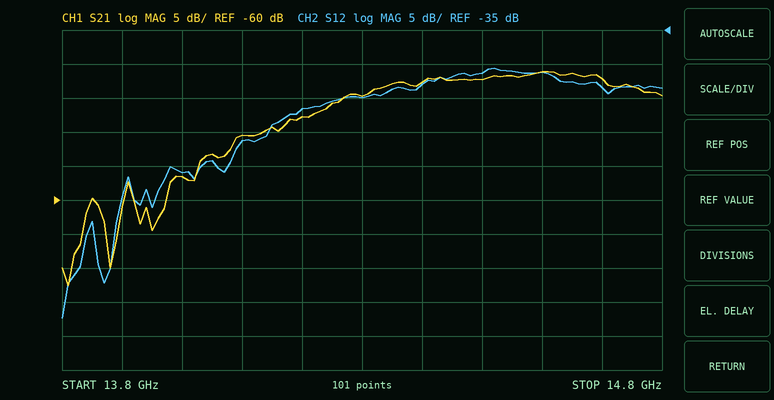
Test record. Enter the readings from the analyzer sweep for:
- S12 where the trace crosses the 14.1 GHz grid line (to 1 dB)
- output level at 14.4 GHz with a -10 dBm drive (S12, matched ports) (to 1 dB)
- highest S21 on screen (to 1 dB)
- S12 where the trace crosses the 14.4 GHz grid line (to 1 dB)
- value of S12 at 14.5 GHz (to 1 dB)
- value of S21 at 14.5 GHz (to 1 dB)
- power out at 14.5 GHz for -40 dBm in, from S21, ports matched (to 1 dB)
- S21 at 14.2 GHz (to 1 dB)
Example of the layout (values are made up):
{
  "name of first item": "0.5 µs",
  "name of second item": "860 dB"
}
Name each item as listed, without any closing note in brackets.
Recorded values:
{
  "S12 where the trace crosses the 14.1 GHz grid line": "-51 dB",
  "output level at 14.4 GHz with a -10 dBm drive (S12, matched ports)": "-53 dBm",
  "highest S21 on screen": "-41 dB",
  "S12 where the trace crosses the 14.4 GHz grid line": "-43 dB",
  "value of S12 at 14.5 GHz": "-41 dB",
  "value of S21 at 14.5 GHz": "-42 dB",
  "power out at 14.5 GHz for -40 dBm in, from S21, ports matched": "-82 dBm",
  "S21 at 14.2 GHz": "-48 dB"
}
